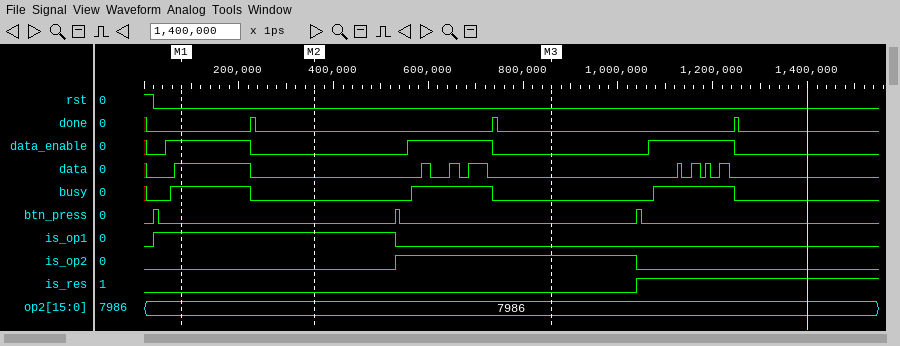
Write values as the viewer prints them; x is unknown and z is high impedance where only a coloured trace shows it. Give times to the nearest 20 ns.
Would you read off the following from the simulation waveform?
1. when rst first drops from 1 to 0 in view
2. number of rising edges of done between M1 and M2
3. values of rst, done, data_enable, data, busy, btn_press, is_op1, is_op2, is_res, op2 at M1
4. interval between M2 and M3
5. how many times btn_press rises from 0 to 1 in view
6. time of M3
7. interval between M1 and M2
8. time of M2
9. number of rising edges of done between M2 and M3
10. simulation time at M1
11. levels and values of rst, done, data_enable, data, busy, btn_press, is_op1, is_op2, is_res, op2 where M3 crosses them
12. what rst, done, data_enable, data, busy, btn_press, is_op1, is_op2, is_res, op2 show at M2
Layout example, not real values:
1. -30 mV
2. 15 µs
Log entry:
1. 20 ns
2. 1
3. rst=0, done=0, data_enable=1, data=1, busy=1, btn_press=0, is_op1=1, is_op2=0, is_res=0, op2=7986
4. 500 ns
5. 3
6. 860 ns
7. 280 ns
8. 360 ns
9. 1
10. 80 ns
11. rst=0, done=0, data_enable=0, data=0, busy=0, btn_press=0, is_op1=0, is_op2=1, is_res=0, op2=7986
12. rst=0, done=0, data_enable=0, data=0, busy=0, btn_press=0, is_op1=1, is_op2=0, is_res=0, op2=7986
